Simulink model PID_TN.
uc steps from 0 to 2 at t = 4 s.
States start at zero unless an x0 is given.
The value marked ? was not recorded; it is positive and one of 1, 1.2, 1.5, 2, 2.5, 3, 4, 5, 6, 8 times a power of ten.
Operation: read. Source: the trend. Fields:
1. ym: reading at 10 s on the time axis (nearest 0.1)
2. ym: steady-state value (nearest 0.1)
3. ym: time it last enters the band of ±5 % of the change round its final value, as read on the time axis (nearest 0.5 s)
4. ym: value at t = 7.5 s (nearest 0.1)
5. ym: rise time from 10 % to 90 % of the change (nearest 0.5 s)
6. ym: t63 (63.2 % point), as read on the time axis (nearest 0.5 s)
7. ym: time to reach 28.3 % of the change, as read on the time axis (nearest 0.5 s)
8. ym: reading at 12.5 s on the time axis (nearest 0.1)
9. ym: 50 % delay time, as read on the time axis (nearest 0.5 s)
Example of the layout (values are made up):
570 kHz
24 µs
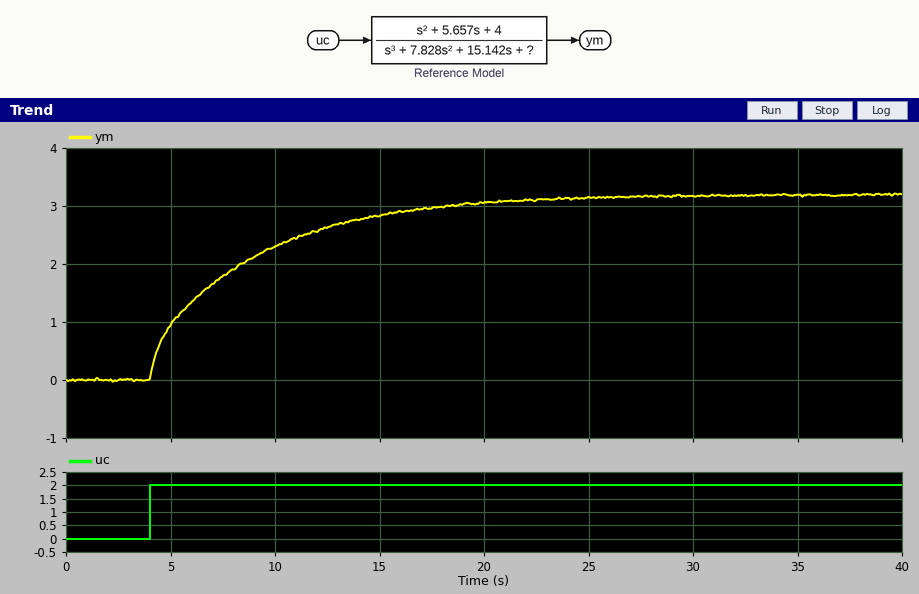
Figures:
2.3
3.2
19.5 s
1.8
11.5 s
8.5 s
5.0 s
2.6
7.0 s
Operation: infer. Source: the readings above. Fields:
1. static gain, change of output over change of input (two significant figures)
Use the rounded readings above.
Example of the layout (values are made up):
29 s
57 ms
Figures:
1.6
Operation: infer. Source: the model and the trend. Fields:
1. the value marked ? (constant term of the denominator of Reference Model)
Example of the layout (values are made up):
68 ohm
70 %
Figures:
2.5
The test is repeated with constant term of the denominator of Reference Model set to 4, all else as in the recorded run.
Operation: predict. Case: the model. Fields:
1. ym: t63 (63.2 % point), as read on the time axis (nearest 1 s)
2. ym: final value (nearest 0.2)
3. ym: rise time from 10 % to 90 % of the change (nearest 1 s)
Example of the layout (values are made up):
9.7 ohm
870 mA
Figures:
6 s
2.0
6 s
